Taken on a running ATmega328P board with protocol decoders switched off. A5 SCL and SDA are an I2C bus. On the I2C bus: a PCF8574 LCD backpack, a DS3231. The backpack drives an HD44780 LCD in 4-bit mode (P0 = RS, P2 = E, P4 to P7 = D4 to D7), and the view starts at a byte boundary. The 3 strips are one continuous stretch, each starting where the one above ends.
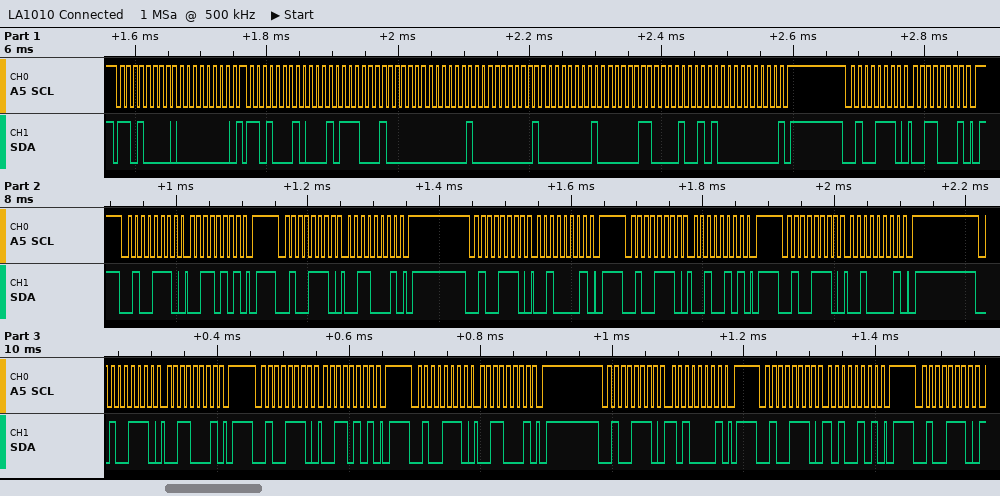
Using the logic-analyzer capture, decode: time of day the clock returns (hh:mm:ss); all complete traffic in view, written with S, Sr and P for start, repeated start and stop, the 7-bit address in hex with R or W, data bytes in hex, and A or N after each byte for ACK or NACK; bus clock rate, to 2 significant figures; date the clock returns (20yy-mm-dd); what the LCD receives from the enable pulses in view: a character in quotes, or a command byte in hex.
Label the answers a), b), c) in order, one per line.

a) 02:20:17
b) S 68W A 00 A Sr 68R A 17 A 20 A 02 A 01 A 01 A 06 A 25 A 00 N P S 27W A 31 A P S 27W A 35 A P S 27W A 31 A P S 27W A 21 A P S 27W A 25 A P S 27W A 21 A P S 27W A 31 A P S 27W A 35 A P S 27W A 31 A P S 27W A A1 A P S 27W A A5 A P S 27W A
c) 100 kHz
d) 2025-06-01
e) '2'
